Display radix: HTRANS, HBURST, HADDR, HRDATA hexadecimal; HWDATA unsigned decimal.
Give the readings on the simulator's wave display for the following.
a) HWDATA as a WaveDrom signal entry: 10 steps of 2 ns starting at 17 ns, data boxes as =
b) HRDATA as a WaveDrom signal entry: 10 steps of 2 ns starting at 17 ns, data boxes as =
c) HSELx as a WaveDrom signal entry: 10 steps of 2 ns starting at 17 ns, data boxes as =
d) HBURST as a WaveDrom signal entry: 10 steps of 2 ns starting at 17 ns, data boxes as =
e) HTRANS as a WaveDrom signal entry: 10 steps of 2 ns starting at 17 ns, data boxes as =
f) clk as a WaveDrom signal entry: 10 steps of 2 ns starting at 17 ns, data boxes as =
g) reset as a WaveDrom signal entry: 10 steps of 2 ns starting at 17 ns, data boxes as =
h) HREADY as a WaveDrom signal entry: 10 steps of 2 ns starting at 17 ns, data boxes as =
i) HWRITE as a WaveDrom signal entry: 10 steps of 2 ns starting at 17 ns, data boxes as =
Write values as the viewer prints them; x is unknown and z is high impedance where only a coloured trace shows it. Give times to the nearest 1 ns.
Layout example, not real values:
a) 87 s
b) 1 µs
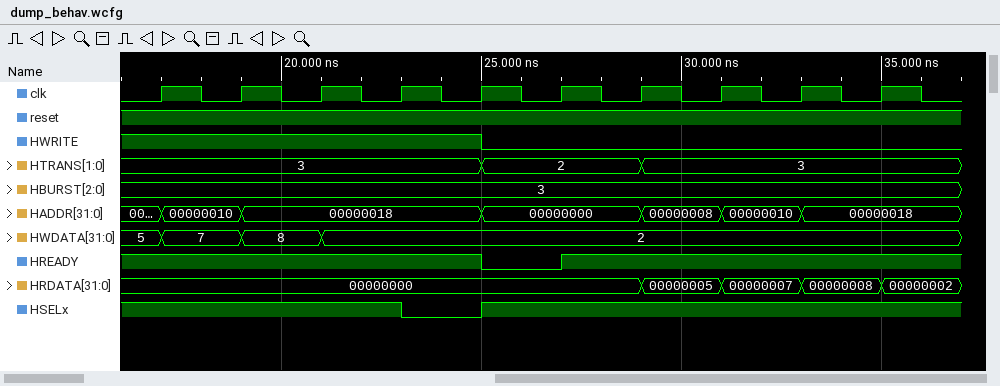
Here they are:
a) {name: 'HWDATA', wave: '===.......', data: '7 8 2'}
b) {name: 'HRDATA', wave: '=.....====', data: '00000000 00000005 00000007 00000008 00000002'}
c) {name: 'HSELx', wave: '1..01.....'}
d) {name: 'HBURST', wave: '=.........', data: '3'}
e) {name: 'HTRANS', wave: '=...=.=...', data: '3 2 3'}
f) {name: 'clk', wave: 'p.........'}
g) {name: 'reset', wave: '1.........'}
h) {name: 'HREADY', wave: '1...01....'}
i) {name: 'HWRITE', wave: '1...0.....'}
